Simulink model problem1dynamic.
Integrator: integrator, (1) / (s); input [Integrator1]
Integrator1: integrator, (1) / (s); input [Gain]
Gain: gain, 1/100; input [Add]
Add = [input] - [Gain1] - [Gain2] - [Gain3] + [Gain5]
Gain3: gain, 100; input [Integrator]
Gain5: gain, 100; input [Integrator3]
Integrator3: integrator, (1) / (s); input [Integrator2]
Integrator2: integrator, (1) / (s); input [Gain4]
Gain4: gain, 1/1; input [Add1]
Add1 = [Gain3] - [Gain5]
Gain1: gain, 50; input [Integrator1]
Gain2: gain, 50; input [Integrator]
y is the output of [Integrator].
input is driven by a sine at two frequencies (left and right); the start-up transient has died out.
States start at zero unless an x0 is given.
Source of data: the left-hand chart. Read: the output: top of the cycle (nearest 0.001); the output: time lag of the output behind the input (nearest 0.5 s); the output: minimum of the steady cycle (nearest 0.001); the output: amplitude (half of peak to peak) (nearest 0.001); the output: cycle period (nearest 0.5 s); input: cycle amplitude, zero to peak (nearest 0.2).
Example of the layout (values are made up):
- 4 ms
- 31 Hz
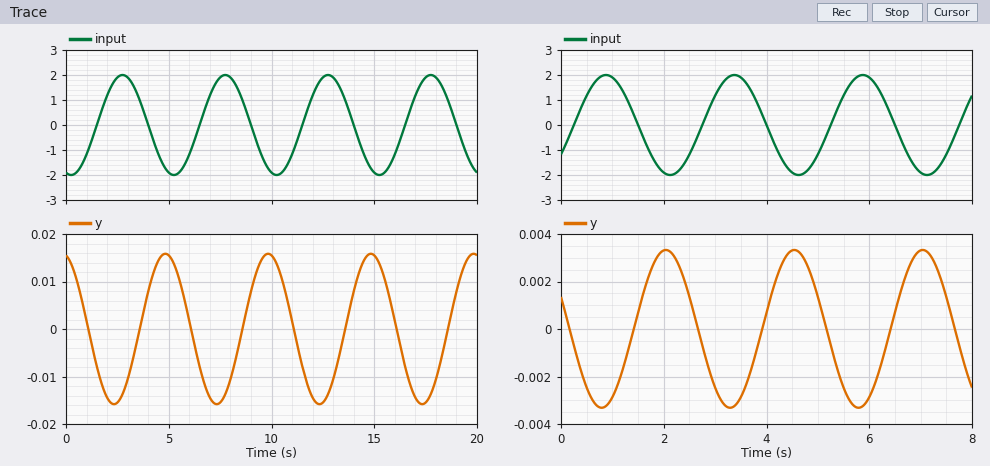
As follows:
- 0.016
- 2.0 s
- -0.016
- 0.016
- 5.0 s
- 2.0
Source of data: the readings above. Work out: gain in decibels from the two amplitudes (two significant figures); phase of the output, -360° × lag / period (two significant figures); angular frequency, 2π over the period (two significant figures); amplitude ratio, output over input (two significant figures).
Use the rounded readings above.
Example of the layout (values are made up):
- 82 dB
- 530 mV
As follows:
- -42 dB
- -140°
- 1.3 rad/s
- 0.0080
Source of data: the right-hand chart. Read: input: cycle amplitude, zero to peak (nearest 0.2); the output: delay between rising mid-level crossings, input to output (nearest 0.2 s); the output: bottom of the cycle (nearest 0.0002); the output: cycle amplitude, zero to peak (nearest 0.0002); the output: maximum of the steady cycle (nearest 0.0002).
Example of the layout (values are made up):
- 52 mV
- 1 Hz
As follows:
- 2.0
- 1.2 s
- -0.0034
- 0.0034
- 0.0034
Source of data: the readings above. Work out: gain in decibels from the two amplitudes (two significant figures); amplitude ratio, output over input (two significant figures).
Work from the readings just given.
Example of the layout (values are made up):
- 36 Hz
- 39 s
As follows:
- -55 dB
- 0.0017
